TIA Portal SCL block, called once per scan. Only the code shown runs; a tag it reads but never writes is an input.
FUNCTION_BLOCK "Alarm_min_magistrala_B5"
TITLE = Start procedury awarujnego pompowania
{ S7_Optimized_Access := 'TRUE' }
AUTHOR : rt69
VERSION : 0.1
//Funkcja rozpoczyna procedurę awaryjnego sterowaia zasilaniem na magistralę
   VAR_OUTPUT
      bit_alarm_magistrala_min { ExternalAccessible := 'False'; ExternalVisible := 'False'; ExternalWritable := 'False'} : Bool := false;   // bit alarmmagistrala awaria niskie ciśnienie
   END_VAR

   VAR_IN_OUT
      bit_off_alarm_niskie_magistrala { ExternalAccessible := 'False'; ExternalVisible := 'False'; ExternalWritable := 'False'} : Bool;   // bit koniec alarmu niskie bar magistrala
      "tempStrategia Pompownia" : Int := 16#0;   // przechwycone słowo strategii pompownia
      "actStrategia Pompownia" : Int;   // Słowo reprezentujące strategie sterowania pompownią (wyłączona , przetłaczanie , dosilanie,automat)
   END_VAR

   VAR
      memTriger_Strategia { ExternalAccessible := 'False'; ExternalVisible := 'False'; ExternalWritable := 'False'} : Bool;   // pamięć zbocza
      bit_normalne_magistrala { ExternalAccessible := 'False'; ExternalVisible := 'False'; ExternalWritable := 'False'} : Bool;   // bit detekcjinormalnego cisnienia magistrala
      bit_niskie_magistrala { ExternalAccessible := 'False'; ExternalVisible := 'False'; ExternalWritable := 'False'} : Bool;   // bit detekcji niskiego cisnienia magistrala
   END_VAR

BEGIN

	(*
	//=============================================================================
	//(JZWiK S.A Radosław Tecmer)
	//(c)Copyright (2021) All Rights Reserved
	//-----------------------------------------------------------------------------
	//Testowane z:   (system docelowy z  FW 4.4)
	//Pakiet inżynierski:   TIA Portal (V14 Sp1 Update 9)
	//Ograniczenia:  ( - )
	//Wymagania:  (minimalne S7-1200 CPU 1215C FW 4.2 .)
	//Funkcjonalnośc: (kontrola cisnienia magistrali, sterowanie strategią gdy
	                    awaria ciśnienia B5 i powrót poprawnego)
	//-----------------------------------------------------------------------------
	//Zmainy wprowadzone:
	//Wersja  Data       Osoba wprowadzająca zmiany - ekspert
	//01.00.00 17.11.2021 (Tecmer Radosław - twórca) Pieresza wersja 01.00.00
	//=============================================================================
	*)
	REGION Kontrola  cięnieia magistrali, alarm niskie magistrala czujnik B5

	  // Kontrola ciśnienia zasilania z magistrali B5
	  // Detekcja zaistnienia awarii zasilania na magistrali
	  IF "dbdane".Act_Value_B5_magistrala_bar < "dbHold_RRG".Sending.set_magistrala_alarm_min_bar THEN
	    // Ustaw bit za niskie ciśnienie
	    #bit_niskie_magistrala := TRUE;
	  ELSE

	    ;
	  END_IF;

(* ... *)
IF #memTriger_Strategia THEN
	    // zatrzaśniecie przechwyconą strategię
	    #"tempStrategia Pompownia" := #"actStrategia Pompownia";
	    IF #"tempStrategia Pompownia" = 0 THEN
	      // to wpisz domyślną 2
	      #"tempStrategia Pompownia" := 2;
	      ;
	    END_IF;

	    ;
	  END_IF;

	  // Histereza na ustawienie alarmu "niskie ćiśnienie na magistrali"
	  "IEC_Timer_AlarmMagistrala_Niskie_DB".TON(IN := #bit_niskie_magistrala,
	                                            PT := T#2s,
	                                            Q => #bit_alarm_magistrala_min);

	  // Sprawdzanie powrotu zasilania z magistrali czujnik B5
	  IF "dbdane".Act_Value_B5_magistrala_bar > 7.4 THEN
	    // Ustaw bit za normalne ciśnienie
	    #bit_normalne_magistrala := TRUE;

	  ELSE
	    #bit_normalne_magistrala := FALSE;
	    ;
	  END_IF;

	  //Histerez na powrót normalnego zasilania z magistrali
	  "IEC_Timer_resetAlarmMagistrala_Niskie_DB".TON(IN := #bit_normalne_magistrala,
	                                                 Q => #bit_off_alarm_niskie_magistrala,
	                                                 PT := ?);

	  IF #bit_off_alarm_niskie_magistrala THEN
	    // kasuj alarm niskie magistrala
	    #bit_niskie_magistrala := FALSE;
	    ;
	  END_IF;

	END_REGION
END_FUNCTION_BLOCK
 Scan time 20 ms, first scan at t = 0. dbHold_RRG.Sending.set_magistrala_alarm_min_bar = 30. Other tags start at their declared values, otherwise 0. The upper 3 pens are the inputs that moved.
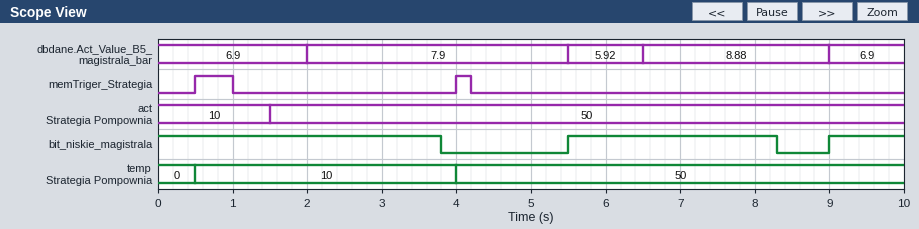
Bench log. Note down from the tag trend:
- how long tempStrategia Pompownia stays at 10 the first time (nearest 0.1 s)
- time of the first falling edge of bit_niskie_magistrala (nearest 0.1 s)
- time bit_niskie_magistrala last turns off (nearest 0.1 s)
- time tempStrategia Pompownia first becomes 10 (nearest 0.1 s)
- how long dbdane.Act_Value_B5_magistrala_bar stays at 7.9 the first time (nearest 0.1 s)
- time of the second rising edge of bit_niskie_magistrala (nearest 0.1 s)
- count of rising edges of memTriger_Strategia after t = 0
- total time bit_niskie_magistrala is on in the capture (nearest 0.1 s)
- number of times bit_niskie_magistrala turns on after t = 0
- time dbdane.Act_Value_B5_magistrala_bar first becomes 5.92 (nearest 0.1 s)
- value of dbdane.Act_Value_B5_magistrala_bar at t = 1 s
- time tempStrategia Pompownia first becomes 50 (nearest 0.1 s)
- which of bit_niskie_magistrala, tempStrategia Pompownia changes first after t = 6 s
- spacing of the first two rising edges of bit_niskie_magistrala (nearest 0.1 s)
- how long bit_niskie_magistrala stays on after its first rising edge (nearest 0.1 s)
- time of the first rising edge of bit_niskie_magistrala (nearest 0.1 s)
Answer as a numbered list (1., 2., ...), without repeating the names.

1. 3.5 s
2. 3.8 s
3. 8.3 s
4. 0.5 s
5. 3.5 s
6. 9.0 s
7. 2
8. 7.6 s
9. 2
10. 5.5 s
11. 6.9
12. 4.0 s
13. bit_niskie_magistrala
14. 3.5 s
15. 2.8 s
16. 5.5 s
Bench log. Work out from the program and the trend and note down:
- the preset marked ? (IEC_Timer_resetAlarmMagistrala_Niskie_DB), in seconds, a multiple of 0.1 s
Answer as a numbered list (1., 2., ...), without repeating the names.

1. 1.8 s
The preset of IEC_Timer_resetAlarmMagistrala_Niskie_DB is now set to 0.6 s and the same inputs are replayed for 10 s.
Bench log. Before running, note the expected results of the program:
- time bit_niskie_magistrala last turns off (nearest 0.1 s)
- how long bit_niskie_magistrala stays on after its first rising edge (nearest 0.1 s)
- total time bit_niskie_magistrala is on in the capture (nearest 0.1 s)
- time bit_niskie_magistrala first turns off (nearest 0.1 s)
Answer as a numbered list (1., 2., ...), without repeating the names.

1. 7.1 s
2. 1.6 s
3. 5.2 s
4. 2.6 s
